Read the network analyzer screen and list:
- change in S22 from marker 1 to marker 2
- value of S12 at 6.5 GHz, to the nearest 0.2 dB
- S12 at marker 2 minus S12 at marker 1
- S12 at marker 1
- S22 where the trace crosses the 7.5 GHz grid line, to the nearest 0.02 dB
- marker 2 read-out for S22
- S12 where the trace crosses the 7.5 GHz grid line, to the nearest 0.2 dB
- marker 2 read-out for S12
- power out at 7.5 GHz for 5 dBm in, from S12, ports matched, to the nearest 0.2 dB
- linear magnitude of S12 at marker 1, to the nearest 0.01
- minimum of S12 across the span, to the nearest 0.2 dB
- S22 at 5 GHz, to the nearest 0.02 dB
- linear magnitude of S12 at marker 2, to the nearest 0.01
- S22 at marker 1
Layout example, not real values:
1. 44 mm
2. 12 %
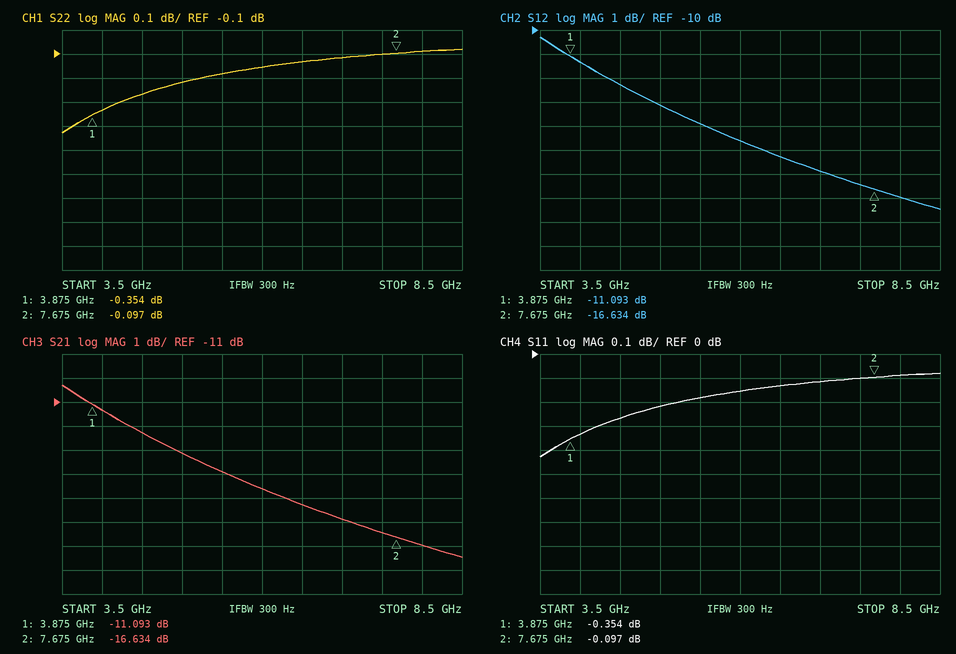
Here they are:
1. 0.257 dB
2. -15.2 dB
3. -5.541 dB
4. -11.093 dB
5. -0.10 dB
6. -0.097 dB
7. -16.4 dB
8. -16.634 dB
9. -11.4 dBm
10. 0.28
11. -17.4 dB
12. -0.22 dB
13. 0.15
14. -0.354 dB
